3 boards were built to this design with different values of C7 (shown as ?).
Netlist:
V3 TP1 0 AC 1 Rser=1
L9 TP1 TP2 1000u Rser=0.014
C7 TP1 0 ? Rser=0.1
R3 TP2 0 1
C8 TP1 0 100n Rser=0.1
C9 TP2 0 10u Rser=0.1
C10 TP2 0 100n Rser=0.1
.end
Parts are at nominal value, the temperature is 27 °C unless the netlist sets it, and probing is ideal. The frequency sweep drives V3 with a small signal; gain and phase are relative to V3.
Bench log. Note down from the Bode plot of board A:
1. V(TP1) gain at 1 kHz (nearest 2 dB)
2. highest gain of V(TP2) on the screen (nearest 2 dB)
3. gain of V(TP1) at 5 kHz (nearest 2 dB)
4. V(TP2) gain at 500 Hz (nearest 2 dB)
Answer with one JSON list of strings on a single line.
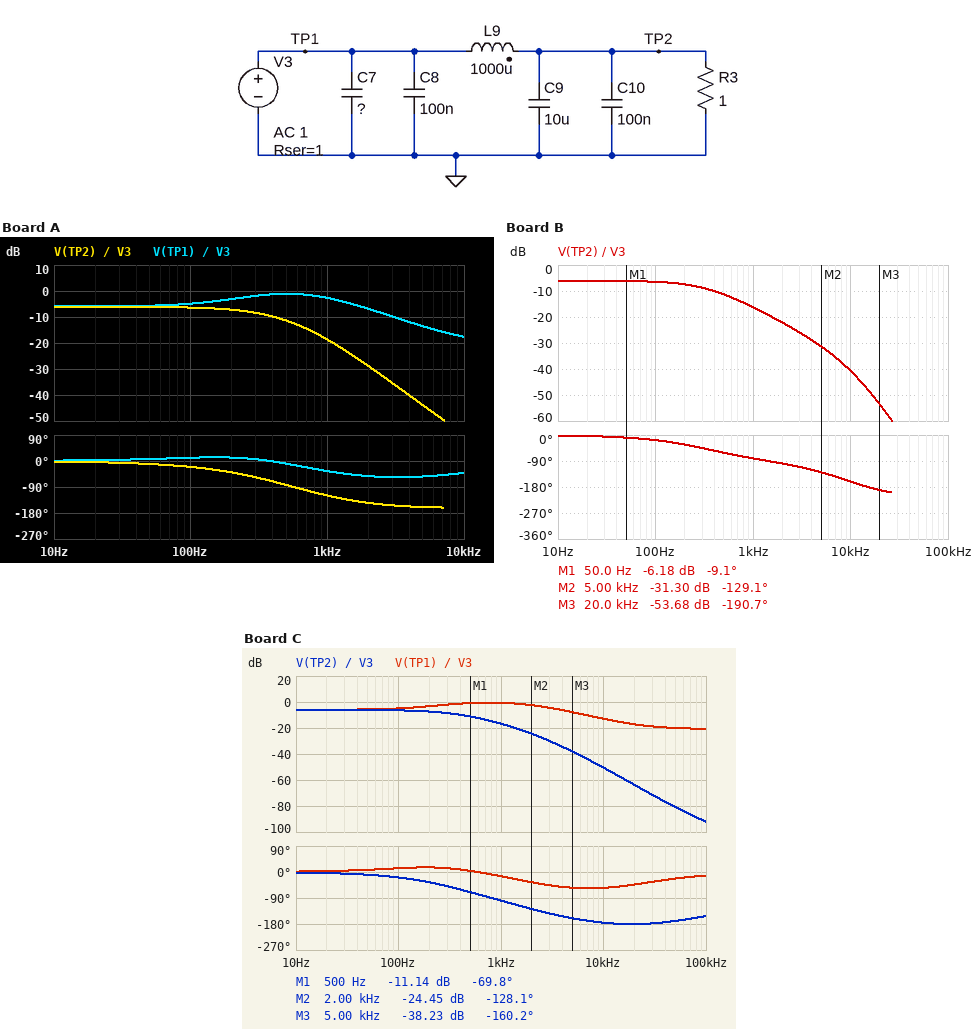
["-2 dB", "-6 dB", "-14 dB", "-12 dB"]
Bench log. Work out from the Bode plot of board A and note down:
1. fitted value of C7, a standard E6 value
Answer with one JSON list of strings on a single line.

["150 µF"]
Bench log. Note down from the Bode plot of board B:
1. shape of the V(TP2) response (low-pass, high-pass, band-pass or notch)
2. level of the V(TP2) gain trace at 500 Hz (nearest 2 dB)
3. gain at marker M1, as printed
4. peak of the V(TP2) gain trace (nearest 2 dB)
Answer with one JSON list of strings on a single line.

["low-pass", "-12 dB", "-6.18 dB", "-6 dB"]
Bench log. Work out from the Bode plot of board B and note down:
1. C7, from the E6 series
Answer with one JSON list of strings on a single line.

["15 µF"]
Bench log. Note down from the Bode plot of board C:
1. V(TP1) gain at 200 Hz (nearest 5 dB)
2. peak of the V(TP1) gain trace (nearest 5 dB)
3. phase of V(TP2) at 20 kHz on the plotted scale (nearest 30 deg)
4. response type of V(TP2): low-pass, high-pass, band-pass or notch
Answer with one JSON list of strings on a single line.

["-5 dB", "0 dB", "-180 deg", "low-pass"]
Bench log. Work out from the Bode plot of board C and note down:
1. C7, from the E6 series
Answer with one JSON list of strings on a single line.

["68 µF"]
